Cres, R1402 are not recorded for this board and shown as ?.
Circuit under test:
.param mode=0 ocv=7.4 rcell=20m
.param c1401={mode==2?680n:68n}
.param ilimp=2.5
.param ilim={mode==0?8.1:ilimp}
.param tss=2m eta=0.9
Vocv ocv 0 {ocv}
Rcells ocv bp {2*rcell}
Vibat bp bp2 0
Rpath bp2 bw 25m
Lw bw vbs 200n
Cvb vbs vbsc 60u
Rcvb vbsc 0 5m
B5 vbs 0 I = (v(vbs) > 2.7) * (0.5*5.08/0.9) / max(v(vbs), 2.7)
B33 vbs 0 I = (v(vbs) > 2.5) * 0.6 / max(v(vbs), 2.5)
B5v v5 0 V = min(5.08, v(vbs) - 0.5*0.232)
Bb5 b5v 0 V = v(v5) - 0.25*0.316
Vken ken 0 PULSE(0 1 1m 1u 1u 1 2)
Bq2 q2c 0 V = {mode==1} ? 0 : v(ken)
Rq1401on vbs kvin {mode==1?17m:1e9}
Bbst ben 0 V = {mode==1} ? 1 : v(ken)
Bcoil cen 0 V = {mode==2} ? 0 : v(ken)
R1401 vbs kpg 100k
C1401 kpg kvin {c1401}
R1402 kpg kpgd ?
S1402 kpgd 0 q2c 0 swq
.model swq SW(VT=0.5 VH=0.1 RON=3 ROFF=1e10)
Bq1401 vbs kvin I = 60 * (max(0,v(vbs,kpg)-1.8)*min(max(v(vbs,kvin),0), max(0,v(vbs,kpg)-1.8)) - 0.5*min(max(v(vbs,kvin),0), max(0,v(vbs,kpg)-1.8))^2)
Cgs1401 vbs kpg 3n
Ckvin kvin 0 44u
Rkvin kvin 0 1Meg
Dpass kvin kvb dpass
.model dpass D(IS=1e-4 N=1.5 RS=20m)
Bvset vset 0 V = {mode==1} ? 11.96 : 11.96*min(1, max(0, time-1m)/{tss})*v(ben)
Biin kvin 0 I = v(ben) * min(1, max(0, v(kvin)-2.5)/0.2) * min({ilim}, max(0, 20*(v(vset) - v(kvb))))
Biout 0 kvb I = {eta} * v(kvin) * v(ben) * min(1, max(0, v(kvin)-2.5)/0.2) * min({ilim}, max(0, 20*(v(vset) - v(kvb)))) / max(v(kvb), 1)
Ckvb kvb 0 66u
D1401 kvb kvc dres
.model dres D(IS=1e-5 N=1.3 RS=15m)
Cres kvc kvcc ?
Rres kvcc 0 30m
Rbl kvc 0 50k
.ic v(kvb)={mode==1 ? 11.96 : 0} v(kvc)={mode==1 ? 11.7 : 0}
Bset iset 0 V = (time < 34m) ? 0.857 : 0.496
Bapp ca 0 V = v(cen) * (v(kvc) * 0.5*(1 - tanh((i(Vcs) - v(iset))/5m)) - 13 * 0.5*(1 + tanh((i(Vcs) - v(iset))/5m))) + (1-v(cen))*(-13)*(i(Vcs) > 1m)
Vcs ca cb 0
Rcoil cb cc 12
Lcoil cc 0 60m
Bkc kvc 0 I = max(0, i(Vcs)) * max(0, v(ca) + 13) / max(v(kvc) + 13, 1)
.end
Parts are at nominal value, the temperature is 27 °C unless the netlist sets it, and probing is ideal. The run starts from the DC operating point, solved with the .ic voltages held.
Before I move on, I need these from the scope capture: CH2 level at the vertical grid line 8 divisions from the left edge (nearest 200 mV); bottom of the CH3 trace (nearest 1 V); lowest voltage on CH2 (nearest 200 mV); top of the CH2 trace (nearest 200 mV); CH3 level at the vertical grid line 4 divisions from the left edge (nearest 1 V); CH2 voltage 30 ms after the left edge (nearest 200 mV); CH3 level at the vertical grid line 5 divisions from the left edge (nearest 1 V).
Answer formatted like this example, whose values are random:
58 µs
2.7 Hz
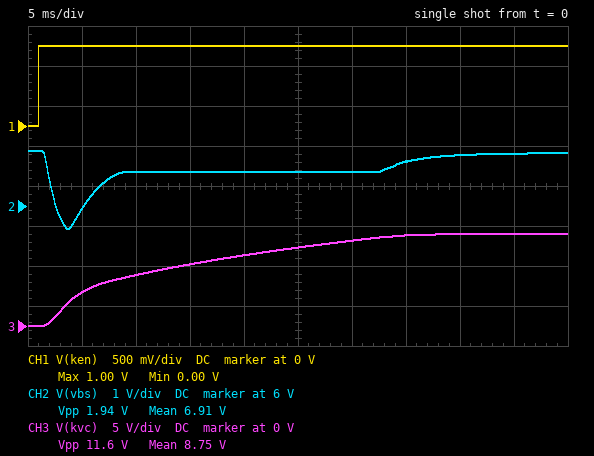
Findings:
7.2 V
0 V
5.4 V
7.4 V
9 V
6.8 V
10 V
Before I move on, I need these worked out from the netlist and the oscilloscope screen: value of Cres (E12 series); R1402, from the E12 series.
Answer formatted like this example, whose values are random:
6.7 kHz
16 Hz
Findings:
22 mF
15 kΩ
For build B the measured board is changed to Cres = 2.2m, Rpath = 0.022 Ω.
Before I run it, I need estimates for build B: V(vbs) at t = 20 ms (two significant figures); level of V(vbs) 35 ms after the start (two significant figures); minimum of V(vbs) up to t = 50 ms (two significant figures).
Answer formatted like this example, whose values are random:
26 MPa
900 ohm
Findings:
7.3 V
7.4 V
6.8 V
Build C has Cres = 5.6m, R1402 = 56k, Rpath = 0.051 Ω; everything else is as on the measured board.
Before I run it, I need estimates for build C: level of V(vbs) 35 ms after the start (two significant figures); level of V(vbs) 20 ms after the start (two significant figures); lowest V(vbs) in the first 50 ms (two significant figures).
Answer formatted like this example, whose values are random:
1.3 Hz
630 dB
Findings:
7.3 V
7.2 V
6.6 V
